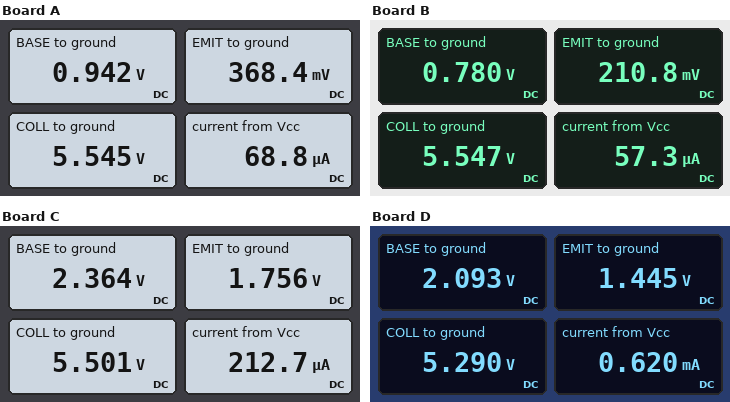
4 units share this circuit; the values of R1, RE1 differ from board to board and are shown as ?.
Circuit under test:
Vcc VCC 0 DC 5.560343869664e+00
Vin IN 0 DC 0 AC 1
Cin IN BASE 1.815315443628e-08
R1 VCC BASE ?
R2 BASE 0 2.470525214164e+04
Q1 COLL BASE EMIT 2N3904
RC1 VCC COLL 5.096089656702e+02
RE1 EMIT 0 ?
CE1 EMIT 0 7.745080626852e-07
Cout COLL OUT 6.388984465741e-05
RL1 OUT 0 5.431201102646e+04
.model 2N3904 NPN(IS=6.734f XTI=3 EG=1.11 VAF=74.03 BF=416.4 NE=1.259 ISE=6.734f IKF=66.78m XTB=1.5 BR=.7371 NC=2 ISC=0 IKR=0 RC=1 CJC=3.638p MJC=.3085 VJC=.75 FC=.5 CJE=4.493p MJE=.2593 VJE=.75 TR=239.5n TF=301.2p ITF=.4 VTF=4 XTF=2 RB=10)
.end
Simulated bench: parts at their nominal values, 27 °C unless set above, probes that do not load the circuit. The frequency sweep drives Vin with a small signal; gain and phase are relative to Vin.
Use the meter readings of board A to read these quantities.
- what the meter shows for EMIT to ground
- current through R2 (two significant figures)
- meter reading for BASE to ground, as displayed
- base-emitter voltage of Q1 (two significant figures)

368.4 mV
38 µA
0.942 V
570 mV
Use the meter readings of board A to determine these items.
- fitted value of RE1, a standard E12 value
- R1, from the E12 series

12 kΩ
120 kΩ
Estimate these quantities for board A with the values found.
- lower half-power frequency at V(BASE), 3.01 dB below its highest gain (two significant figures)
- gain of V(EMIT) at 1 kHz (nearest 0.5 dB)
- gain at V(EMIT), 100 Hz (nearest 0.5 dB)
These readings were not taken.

550 Hz
-14.0 dB
-14.5 dB
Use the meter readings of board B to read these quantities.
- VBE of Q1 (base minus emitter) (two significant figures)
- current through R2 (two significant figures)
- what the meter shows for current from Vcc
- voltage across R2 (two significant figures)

570 mV
32 µA
57.3 µA
780 mV
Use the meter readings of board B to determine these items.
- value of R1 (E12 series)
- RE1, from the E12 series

150 kΩ
8.2 kΩ
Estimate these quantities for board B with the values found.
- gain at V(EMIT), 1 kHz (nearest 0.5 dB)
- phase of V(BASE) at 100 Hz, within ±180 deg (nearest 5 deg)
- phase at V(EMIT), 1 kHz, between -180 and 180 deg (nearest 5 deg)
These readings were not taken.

-15.0 dB
75 deg
-50 deg
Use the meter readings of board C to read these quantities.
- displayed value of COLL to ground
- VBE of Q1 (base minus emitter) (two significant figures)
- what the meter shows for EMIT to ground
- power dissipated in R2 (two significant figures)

5.501 V
610 mV
1.756 V
230 µW
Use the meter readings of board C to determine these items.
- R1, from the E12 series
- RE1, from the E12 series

33 kΩ
15 kΩ
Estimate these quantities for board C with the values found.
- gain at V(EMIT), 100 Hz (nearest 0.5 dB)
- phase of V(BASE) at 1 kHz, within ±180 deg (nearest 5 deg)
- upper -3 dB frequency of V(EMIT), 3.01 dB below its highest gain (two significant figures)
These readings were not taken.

-16.5 dB
35 deg
2.2 kHz
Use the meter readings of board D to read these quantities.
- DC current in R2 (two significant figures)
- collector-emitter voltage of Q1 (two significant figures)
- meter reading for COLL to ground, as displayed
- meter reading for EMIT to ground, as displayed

85 µA
3.8 V
5.290 V
1.445 V
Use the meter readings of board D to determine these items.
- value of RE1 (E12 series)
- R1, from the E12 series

2.7 kΩ
39 kΩ
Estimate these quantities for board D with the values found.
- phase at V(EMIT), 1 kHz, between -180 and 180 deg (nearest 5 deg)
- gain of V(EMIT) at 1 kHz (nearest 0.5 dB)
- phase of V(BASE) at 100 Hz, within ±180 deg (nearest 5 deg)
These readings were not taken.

15 deg
-3.5 dB
80 deg
